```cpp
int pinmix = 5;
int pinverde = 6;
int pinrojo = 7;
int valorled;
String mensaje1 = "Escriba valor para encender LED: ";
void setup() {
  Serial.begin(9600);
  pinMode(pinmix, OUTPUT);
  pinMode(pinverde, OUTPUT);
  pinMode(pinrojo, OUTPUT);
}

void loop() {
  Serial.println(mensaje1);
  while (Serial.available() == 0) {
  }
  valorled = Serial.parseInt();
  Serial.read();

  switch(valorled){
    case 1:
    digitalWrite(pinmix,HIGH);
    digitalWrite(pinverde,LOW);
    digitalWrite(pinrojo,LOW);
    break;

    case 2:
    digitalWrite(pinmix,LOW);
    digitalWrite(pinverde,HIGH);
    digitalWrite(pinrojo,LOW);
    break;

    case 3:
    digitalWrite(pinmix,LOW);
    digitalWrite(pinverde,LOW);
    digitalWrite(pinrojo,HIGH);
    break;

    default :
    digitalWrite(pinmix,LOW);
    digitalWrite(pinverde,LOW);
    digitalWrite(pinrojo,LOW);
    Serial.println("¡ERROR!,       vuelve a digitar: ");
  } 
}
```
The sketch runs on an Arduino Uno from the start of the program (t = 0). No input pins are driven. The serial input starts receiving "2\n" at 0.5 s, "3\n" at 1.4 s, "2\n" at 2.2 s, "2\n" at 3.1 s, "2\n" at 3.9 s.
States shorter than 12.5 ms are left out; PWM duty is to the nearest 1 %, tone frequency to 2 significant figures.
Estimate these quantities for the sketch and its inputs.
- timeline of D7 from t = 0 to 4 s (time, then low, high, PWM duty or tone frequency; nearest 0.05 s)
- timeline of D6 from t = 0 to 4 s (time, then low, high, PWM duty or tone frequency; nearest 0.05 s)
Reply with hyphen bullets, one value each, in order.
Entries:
- 0 s low; 1.4 s high; 2.2 s low
- 0 s low; 0.5 s high; 1.4 s low; 2.2 s high
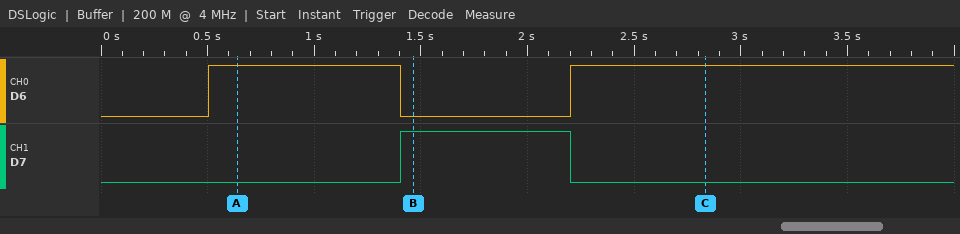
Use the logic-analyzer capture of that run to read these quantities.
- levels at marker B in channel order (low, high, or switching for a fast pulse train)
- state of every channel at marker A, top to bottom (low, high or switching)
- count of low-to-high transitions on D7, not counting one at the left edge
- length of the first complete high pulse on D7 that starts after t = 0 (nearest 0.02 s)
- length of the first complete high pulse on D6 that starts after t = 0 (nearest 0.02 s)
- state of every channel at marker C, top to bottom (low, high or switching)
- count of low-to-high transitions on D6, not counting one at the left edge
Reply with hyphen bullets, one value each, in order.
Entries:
- D6 low, D7 high
- D6 high, D7 low
- 1
- 0.80 s
- 0.90 s
- D6 high, D7 low
- 2
